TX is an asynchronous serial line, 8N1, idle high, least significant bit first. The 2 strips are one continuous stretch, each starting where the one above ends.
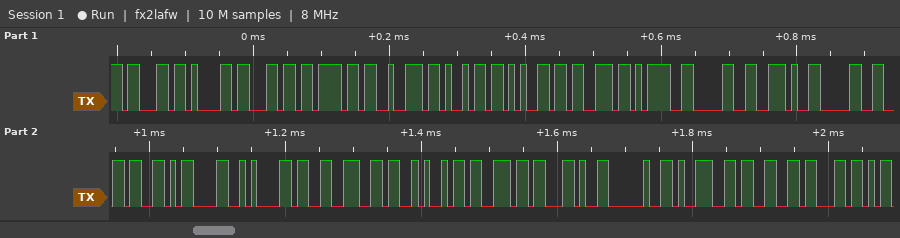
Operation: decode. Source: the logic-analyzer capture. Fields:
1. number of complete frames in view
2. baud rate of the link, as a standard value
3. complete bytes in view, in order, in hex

24
115200 baud
63 61 6C 6F 72 69 65 73 3D 30 2E 30 36 0D 0A 33 36 69 6E 2C 20 39 33 63
